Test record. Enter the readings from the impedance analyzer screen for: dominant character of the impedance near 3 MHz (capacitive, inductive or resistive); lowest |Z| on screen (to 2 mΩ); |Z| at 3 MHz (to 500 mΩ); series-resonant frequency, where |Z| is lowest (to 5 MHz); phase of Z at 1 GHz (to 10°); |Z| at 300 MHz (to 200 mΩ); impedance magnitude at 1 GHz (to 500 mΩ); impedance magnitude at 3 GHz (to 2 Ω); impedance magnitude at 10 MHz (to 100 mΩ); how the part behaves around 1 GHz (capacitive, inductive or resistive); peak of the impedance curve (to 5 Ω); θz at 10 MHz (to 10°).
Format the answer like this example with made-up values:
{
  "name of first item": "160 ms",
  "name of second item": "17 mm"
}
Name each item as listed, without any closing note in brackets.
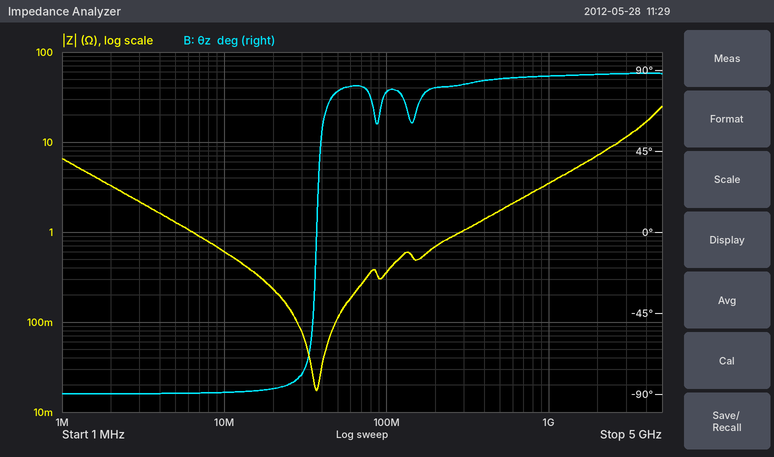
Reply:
{
  "dominant character of the impedance near 3 MHz": "capacitive",
  "lowest |Z| on screen": "18 mΩ",
  "|Z| at 3 MHz": "2.0 Ω",
  "series-resonant frequency, where |Z| is lowest": "35 MHz",
  "phase of Z at 1 GHz": "90°",
  "|Z| at 300 MHz": "1.0 Ω",
  "impedance magnitude at 1 GHz": "3.5 Ω",
  "impedance magnitude at 3 GHz": "12 Ω",
  "impedance magnitude at 10 MHz": "600 mΩ",
  "how the part behaves around 1 GHz": "inductive",
  "peak of the impedance curve": "25 Ω",
  "θz at 10 MHz": "-90°"
}
